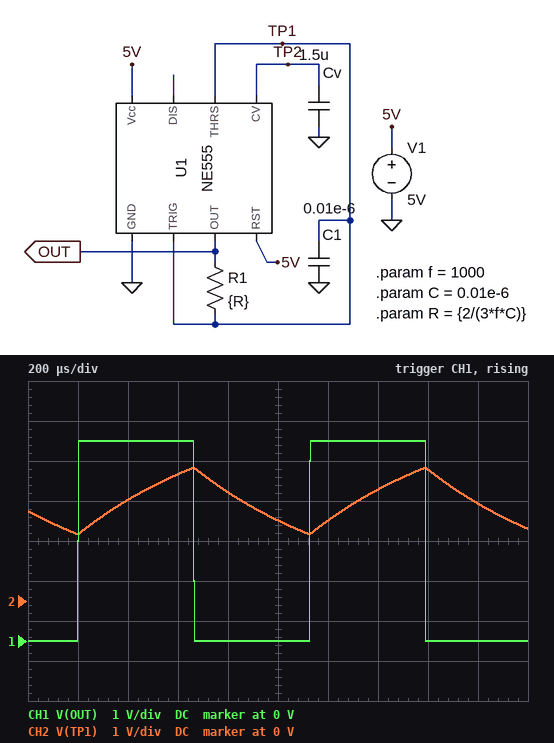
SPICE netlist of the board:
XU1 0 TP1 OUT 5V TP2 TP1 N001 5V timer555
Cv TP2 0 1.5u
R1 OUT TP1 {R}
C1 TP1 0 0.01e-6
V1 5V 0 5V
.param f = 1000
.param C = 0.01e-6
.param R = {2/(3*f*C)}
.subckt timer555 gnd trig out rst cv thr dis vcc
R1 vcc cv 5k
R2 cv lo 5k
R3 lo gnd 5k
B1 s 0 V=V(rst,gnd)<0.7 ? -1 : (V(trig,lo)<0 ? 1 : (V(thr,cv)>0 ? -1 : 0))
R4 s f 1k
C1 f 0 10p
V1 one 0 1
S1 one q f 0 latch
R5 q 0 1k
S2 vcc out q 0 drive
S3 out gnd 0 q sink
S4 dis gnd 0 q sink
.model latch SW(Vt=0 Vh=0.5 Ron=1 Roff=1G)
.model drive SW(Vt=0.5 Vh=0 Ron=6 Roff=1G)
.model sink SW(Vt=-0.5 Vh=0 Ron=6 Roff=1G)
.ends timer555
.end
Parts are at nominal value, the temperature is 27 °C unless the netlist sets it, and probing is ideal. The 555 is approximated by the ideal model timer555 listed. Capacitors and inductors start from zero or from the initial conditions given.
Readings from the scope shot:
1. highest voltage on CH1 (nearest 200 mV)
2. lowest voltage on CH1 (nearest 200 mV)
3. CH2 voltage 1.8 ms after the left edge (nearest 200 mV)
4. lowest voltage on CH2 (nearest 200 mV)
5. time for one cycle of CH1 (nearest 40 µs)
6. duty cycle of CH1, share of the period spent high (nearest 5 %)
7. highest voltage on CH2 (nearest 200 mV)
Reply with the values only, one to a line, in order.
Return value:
5.0 V
0 V
2.4 V
1.6 V
920 µs
50 %
3.4 V
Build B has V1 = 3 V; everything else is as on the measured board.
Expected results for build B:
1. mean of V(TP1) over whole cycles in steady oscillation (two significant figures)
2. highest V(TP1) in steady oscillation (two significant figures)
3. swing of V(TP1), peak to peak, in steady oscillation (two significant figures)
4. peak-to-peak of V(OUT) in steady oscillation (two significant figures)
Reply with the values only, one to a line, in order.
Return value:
1.5 V
2.0 V
1.0 V
3.0 V
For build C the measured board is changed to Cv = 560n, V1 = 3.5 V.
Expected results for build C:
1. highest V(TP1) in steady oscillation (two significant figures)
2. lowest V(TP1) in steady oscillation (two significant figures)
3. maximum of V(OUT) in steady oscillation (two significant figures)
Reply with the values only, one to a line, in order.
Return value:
2.3 V
1.2 V
3.5 V
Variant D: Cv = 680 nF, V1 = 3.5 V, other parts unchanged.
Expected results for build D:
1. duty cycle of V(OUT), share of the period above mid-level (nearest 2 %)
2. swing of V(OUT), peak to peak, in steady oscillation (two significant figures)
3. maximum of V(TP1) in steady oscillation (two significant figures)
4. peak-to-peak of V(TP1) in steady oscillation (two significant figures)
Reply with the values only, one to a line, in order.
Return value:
50 %
3.5 V
2.3 V
1.2 V
